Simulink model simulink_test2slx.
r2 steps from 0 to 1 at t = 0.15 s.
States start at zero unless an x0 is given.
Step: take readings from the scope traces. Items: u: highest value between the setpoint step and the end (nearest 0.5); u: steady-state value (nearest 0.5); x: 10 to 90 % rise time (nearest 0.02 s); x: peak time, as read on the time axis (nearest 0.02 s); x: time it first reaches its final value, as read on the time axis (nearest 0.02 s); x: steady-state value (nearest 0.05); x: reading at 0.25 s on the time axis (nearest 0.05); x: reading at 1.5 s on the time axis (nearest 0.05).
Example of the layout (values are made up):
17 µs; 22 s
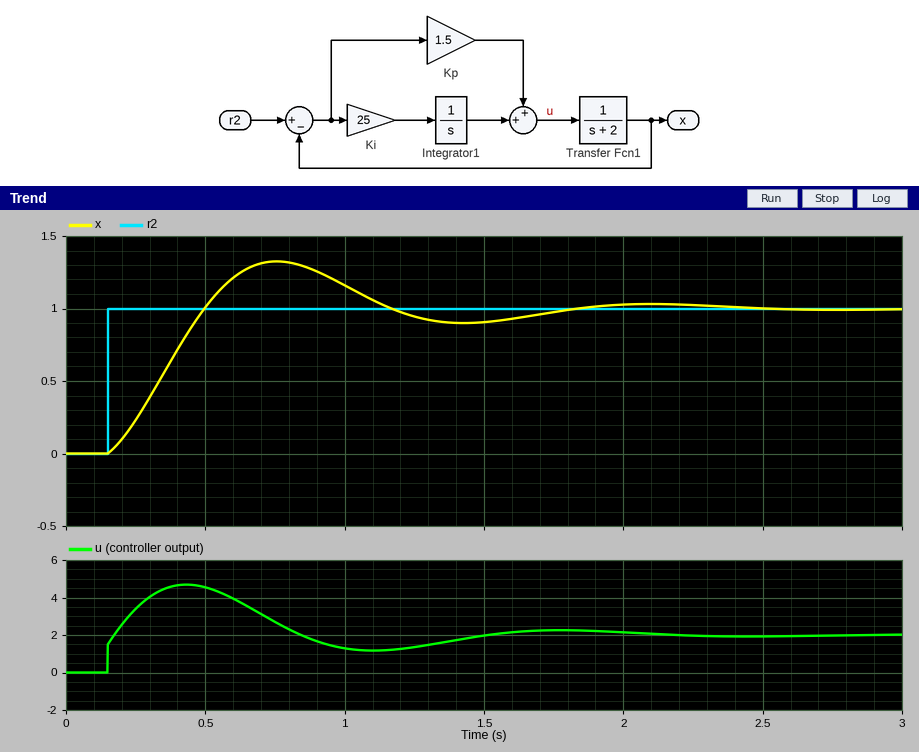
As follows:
4.5; 2.0; 0.26 s; 0.76 s; 0.50 s; 1.00; 0.25; 0.90
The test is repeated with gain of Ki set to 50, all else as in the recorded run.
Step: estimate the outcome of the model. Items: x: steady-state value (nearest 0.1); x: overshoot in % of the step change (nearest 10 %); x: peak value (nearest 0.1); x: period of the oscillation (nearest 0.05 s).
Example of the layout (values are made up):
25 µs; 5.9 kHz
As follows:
1.0; 50 %; 1.5; 0.90 s
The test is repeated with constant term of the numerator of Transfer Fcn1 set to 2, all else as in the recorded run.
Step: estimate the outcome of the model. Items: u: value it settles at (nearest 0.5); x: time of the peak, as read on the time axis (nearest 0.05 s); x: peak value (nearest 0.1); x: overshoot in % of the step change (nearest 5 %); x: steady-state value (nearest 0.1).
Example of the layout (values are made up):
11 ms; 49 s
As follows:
1.0; 0.55 s; 1.3; 35 %; 1.0
